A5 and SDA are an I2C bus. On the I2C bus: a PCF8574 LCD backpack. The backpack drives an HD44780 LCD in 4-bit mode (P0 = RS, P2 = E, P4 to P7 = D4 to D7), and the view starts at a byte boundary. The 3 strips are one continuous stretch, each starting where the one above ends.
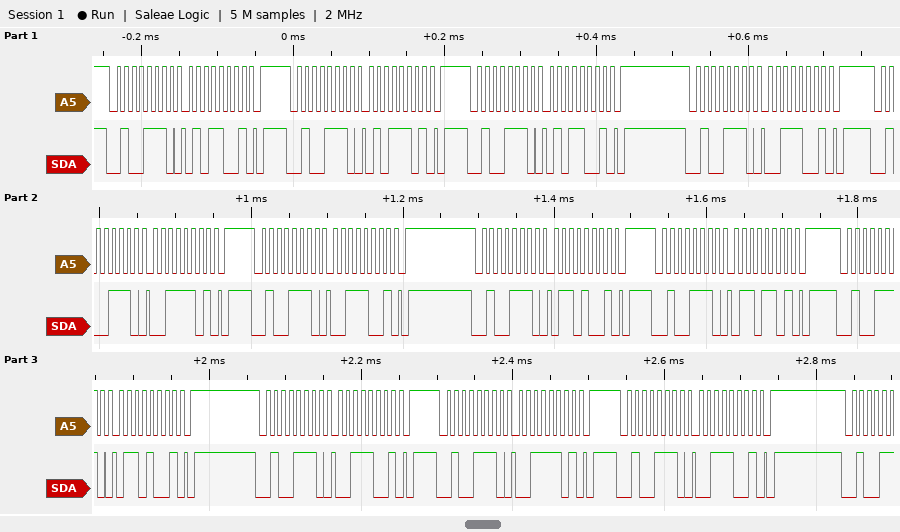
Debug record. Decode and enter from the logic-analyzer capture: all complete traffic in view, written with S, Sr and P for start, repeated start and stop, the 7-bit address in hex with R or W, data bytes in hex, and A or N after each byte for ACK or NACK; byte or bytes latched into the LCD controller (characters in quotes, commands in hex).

S 27W A 59 A P S 27W A 5D A P S 27W A 59 A P S 27W A 39 A P S 27W A 3D A P S 27W A 39 A P S 27W A 69 A P S 27W A 6D A P S 27W A 69 A P S 27W A 39 A P S 27W A 3D A P S 27W A 39 A P
'S' 'c'
